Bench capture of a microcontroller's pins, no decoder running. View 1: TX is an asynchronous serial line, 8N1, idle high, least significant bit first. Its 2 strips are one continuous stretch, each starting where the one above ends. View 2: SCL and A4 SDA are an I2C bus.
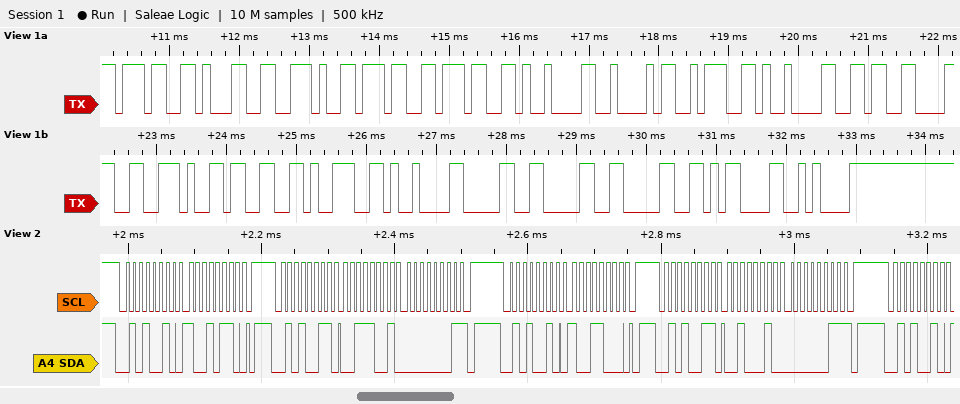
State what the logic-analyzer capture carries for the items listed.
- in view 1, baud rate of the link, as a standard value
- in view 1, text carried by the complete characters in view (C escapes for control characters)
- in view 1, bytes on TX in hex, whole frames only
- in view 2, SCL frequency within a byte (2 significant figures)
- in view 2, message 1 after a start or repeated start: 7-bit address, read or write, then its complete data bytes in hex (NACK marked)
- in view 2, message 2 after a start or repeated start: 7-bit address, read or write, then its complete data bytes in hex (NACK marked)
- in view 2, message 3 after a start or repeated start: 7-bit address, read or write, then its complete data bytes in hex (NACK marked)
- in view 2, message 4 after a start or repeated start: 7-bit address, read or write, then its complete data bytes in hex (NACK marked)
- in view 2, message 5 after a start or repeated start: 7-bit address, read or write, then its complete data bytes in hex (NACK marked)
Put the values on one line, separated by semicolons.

9600 baud; "71.77\tB:\t68.39\t000\r\n"; 0x37 0x31 0x2E 0x37 0x37 0x09 0x42 0x3A 0x09 0x36 0x38 0x2E 0x33 0x39 0x09 0x30 0x30 0x30 0x0D 0x0A; 100 kHz; 0x29 write: 96; 0x29 read: 39 01 NACK; 0x29 write: 98; 0x29 read: 22 03 NACK; 0x29 write
